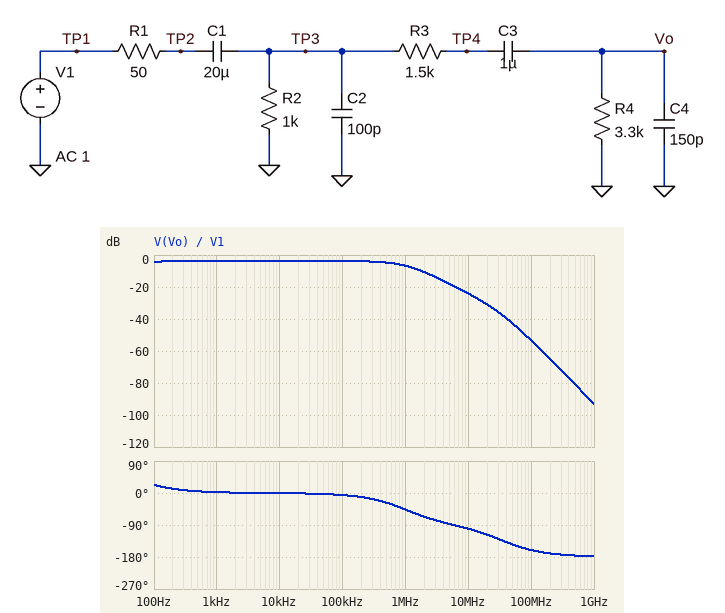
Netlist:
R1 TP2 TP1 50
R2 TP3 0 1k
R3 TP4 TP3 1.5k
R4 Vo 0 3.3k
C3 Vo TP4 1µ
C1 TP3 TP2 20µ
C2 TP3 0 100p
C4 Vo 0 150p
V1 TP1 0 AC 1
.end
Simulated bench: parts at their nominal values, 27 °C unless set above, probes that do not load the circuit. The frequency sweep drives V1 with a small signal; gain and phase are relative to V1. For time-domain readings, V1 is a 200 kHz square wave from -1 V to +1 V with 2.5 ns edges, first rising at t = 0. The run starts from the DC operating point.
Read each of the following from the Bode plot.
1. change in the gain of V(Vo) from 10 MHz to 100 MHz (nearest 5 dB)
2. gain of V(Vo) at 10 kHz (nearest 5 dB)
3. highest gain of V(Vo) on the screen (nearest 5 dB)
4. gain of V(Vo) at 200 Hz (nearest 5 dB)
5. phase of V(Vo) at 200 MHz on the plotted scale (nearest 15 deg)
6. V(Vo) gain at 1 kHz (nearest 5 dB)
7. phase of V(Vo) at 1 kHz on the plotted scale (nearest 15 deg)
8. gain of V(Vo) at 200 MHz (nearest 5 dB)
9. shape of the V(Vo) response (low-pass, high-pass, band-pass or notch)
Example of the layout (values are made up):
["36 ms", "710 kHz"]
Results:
["-30 dB", "-5 dB", "-5 dB", "-5 dB", "-165 deg", "-5 dB", "0 deg", "-65 dB", "low-pass"]
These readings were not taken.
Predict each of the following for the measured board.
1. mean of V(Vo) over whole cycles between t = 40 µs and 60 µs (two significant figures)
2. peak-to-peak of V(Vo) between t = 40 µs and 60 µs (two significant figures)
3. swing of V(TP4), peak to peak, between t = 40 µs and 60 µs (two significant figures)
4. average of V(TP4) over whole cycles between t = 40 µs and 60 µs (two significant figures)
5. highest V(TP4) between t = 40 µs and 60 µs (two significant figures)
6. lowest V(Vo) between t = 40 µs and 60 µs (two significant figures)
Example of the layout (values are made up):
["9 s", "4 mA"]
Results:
["640 mV", "1.3 V", "1.3 V", "650 mV", "1.3 V", "-10 mV"]
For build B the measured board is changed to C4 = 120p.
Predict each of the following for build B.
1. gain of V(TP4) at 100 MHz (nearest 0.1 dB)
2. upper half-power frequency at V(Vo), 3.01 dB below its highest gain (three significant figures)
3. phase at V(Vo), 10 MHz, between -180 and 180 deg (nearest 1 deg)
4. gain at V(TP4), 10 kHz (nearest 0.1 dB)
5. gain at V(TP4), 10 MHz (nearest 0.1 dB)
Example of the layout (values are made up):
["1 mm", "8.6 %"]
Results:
["-51.5 dB", "1.26 MHz", "-99 deg", "-3.8 dB", "-22.2 dB"]
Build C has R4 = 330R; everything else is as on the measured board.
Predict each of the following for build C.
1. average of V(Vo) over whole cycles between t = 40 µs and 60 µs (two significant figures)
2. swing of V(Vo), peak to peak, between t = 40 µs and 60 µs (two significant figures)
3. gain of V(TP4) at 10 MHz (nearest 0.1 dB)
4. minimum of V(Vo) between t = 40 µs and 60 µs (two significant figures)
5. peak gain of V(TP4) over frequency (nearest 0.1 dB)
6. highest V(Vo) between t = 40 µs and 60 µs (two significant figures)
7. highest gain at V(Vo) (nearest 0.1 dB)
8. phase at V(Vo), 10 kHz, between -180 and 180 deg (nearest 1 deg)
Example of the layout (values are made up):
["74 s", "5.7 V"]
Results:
["160 mV", "340 mV", "-24.7 dB", "-6.0 mV", "-1.5 dB", "330 mV", "-15.5 dB", "0 deg"]
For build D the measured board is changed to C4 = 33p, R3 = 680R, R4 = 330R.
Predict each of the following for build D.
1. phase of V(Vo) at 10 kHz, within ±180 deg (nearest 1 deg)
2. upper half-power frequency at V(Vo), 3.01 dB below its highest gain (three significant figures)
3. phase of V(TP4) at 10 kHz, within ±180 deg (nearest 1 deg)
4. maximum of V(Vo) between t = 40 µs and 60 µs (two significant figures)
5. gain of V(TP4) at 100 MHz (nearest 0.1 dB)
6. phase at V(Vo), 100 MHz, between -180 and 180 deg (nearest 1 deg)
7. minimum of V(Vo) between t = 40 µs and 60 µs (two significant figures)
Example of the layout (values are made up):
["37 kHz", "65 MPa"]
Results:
["1 deg", "16.7 MHz", "-2 deg", "580 mV", "-33.7 dB", "-148 deg", "-18 mV"]
